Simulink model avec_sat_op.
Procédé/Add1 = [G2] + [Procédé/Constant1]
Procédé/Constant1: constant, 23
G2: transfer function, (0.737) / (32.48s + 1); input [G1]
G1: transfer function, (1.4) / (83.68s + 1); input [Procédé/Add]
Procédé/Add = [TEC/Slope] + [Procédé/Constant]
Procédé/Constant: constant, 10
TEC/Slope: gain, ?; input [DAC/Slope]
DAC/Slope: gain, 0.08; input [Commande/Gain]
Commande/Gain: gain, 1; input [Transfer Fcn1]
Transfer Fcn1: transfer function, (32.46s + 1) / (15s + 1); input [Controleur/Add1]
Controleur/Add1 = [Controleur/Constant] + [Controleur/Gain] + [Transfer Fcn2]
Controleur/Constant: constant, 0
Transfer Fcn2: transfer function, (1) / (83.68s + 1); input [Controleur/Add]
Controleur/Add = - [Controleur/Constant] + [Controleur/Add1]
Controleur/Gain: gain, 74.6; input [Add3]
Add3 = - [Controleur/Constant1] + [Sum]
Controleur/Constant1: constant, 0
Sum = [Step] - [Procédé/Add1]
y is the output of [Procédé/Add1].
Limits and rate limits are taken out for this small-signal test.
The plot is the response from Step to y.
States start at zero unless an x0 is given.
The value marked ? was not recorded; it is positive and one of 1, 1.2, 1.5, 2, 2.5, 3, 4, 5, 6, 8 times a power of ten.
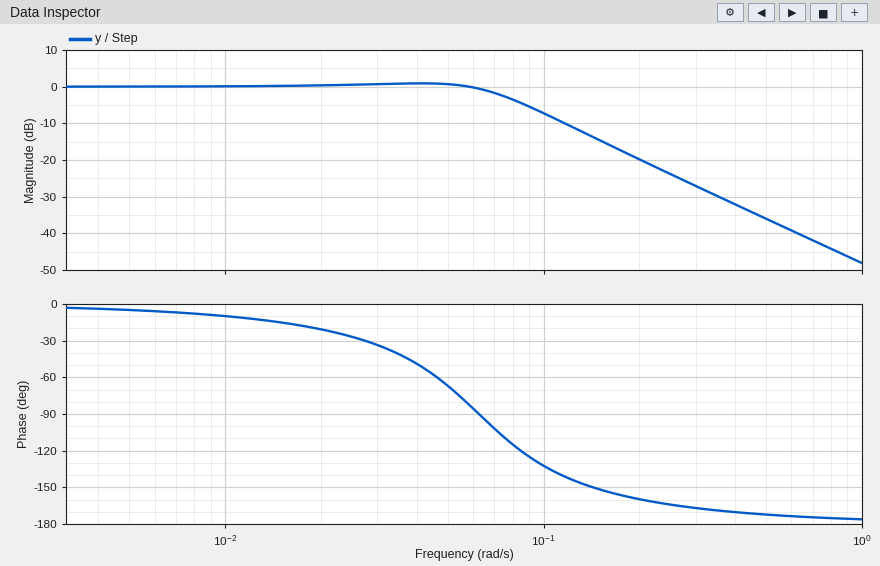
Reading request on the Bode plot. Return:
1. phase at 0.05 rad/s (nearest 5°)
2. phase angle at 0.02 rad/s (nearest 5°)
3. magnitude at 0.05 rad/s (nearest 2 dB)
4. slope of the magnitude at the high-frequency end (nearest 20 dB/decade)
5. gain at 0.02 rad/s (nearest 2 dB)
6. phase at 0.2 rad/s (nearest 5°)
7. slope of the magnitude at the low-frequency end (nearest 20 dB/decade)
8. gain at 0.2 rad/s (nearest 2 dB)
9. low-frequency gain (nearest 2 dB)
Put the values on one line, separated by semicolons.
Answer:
-65°; -20°; 0 dB; -40 dB/decade; 0 dB; -160°; 0 dB/decade; -20 dB; 0 dB
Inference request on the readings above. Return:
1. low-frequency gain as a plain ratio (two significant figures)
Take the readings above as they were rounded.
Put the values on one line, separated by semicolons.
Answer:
1.0
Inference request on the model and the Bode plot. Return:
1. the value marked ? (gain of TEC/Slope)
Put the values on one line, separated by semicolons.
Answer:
0.8
